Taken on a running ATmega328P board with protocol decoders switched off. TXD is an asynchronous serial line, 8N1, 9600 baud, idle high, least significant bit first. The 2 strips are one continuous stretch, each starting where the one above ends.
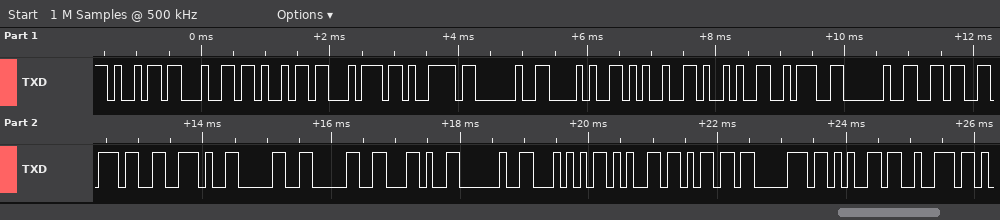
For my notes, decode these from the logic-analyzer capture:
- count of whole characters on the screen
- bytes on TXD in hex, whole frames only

24
69 64 69 74 79 20 28 25 29 3A 20 36 37 2E 30 30 2C 20 54 65 6D 70 65 72
